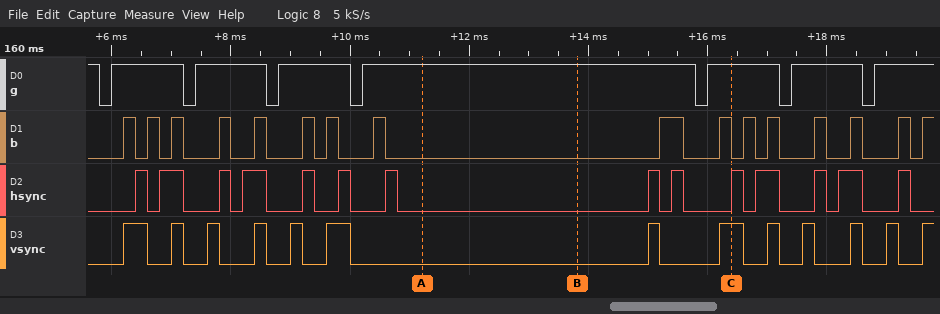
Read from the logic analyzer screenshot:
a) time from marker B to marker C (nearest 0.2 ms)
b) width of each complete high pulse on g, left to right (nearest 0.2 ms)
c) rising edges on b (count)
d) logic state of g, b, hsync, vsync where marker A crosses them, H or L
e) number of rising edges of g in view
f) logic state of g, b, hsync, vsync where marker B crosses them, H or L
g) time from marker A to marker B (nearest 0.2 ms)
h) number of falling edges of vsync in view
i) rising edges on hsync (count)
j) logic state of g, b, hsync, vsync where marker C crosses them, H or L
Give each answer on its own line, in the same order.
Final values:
2.6 ms
1.2 ms, 1.2 ms, 1.2 ms, 5.6 ms, 1.2 ms, 1.2 ms
16
g=H, b=L, hsync=L, vsync=L
7
g=H, b=L, hsync=L, vsync=L
2.6 ms
12
14
g=H, b=L, hsync=H, vsync=H
